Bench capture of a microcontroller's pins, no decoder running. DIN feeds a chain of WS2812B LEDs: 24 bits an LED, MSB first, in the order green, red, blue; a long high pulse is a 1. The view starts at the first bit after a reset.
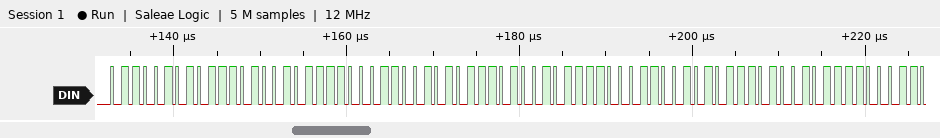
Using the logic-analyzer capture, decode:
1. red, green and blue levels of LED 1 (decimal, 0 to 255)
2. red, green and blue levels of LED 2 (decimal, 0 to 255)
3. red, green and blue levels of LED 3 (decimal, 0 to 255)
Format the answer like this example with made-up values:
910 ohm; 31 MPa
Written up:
116, 101, 188; 116, 101, 188; 116, 101, 188
